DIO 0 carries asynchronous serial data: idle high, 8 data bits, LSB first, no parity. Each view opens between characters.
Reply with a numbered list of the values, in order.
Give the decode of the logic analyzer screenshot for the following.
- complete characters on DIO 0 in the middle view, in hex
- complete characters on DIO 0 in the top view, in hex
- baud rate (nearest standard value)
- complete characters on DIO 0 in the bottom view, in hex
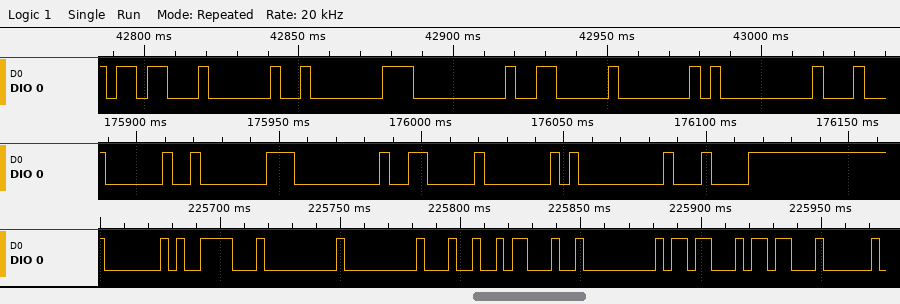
1. 20, C0, 00, 06, 40, 00, 84
2. 1B, 20, C0, 00, 06, 40, 00
3. 300 baud
4. 40, 1E, 00, 00, 24, 23, 00, 1B, 1B
